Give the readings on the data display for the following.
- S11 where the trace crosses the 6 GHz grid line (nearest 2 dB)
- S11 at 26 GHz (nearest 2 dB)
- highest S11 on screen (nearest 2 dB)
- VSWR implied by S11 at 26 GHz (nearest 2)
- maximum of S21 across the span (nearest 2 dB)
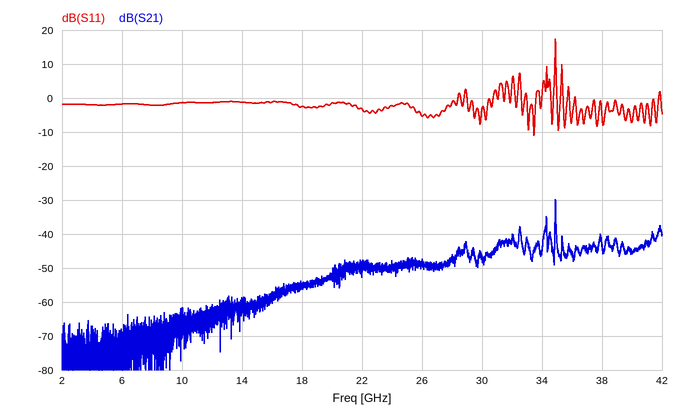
-2 dB
-6 dB
18 dB
4
-30 dB
